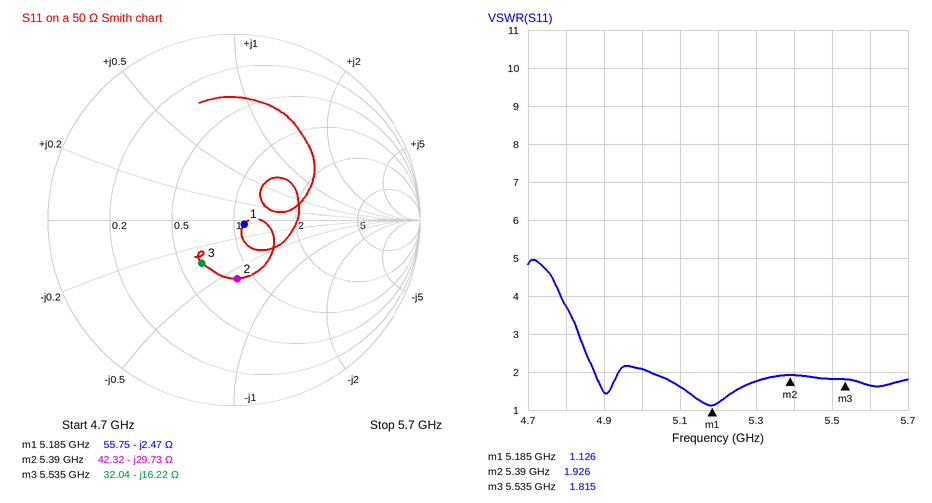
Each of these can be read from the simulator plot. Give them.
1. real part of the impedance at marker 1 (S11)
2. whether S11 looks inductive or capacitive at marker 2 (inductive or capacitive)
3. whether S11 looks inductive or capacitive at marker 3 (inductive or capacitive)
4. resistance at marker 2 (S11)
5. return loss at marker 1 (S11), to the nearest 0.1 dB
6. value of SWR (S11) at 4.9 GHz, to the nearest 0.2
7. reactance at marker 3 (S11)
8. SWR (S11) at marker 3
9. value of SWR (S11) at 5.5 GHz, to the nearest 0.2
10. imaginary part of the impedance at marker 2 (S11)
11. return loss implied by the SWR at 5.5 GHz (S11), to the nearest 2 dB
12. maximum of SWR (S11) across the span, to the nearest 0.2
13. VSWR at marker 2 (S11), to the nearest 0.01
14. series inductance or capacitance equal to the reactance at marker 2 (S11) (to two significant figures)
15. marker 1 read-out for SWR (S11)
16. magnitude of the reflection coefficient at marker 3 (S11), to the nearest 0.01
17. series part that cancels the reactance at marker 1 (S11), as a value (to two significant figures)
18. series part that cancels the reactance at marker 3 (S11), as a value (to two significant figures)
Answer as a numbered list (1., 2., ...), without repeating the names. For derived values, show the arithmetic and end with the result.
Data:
1. 55.75 Ω
2. capacitive
3. capacitive
4. 42.32 Ω
5. 24.6 dB
6. 1.4
7. -16.22 Ω
8. 1.815
9. 1.8
10. -29.73 Ω
11. −20 log10((1.8 − 1)/(1.8 + 1)) ≈ 10.9 dB, so 10 dB to the nearest 2 dB
12. 5.0
13. 1.93
14. C = 1/(2π × 5.39 GHz × 29.73 Ω) ≈ 993 fF, so 990 fF to two significant figures
15. 1.126
16. 0.29
17. L = 2.47 Ω/(2π × 5.185 GHz) ≈ 76 pH
18. L = 16.22 Ω/(2π × 5.535 GHz) ≈ 466 pH, so 470 pH to two significant figures
